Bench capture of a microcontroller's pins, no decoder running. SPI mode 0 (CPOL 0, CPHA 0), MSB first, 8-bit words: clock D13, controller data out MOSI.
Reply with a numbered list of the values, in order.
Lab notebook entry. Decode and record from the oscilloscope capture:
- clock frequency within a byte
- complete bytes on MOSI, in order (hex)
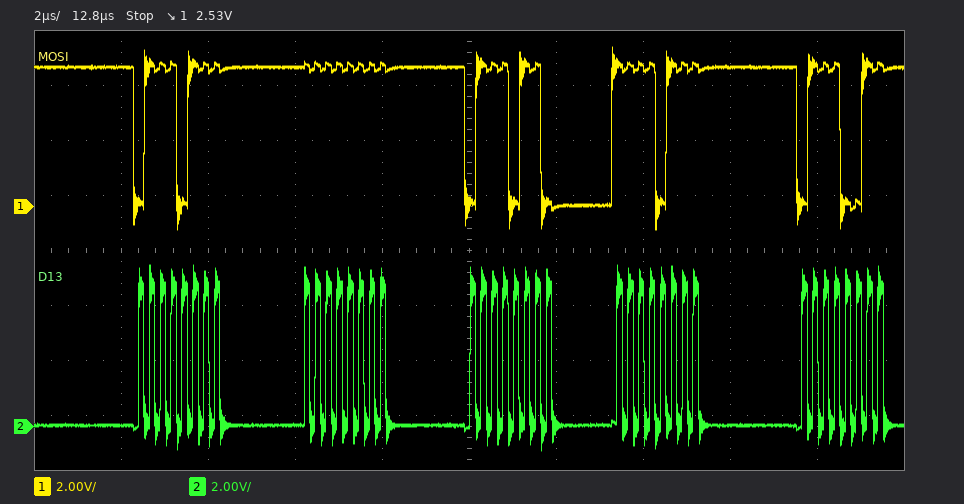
1. 4 MHz
2. 77 FF 76 F7 73
